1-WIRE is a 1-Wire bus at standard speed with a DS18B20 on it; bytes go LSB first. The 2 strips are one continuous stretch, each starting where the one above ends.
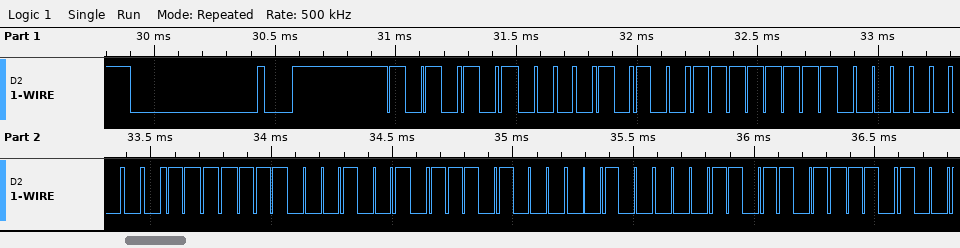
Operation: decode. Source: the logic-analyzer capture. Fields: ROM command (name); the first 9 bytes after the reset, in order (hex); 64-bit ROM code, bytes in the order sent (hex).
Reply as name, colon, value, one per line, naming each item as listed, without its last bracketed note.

ROM command: Match ROM
the first 9 bytes after the reset, in order: 55 28 FF 00 FE 48 17 04 DB
64-bit ROM code, bytes in the order sent: 28 FF 00 FE 48 17 04 DB
